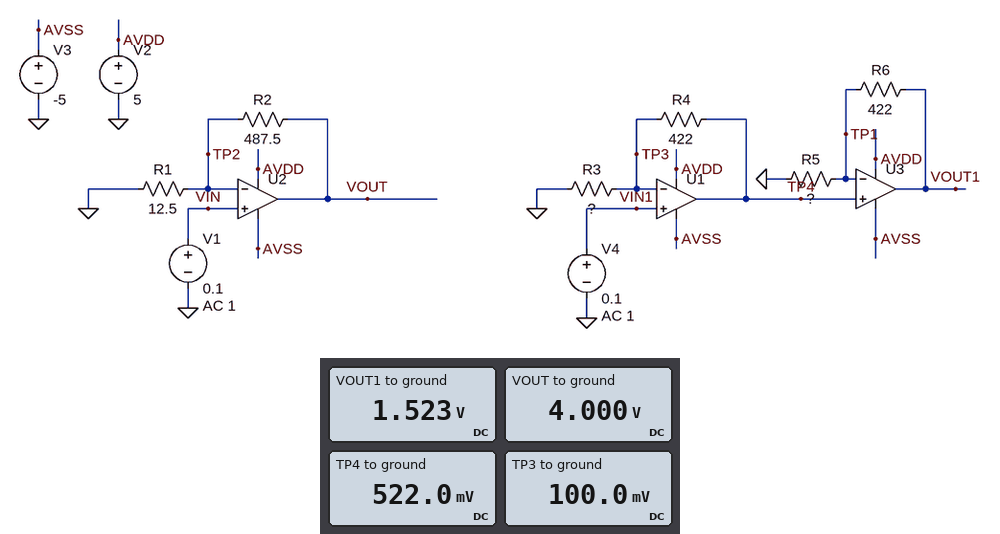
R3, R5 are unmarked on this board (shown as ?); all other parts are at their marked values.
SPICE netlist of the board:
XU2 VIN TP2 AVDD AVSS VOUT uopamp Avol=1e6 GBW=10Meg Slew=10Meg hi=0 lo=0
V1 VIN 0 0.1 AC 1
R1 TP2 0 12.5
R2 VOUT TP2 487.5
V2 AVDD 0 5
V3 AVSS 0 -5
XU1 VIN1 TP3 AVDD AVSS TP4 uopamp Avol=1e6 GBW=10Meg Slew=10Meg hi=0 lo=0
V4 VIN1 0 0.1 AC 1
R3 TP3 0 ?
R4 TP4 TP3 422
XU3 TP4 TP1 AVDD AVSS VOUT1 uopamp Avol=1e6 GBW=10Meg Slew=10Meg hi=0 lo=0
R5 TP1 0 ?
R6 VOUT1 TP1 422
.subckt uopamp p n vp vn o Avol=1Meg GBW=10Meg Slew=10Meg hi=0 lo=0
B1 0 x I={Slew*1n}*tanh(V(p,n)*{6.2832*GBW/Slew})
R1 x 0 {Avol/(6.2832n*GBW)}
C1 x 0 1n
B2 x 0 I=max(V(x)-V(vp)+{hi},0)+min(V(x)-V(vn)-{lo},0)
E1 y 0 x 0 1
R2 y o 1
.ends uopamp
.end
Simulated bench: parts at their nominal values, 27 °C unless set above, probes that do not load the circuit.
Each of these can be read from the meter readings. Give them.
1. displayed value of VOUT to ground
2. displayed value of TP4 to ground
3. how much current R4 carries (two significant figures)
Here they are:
4.000 V
522.0 mV
1.0 mA
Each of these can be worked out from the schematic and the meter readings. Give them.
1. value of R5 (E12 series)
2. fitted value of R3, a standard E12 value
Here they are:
220 Ω
100 Ω
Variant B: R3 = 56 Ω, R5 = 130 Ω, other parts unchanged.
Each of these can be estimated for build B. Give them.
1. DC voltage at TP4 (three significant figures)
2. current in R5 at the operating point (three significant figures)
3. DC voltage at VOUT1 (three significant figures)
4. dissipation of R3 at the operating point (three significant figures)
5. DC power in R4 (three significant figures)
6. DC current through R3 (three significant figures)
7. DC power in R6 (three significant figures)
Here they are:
854 mV
6.57 mA
3.62 V
179 µW
1.35 mW
1.79 mA
18.2 mW
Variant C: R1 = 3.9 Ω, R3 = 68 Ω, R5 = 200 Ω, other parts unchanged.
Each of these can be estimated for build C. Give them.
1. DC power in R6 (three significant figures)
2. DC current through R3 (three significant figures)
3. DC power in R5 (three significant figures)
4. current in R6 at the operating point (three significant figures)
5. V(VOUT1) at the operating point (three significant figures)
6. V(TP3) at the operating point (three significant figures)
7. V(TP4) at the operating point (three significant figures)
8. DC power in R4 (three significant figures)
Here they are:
5.48 mW
1.47 mA
2.60 mW
3.60 mA
2.24 V
100 mV
721 mV
913 µW
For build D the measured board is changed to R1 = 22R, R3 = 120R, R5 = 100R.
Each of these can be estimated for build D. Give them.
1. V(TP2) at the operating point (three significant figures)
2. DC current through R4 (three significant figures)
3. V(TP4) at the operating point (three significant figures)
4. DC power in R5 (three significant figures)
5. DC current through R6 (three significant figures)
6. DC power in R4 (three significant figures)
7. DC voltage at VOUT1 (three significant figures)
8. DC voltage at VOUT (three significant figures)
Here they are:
100 mV
833 µA
452 mV
2.04 mW
4.52 mA
293 µW
2.36 V
2.32 V
